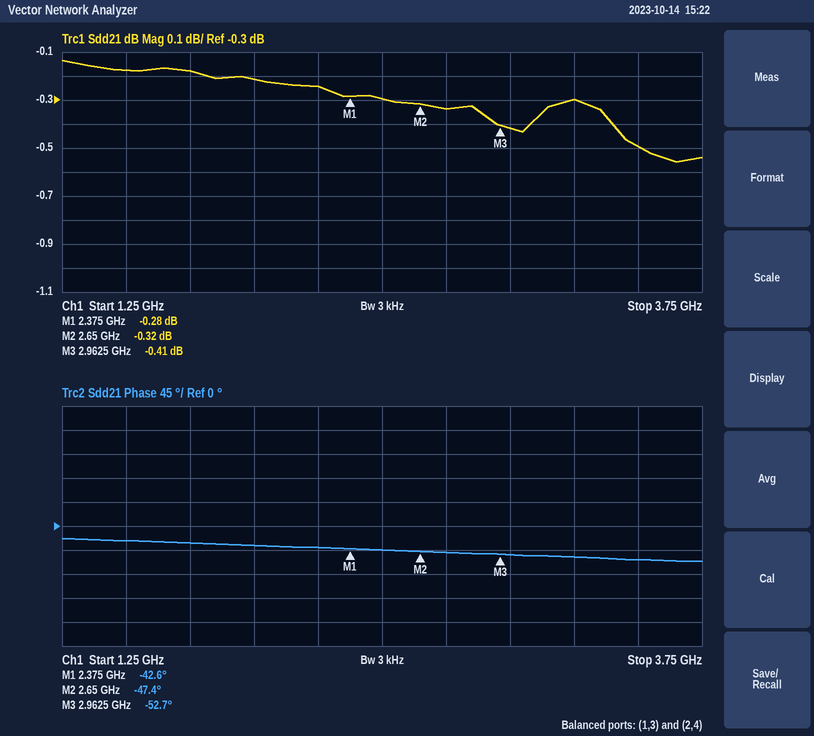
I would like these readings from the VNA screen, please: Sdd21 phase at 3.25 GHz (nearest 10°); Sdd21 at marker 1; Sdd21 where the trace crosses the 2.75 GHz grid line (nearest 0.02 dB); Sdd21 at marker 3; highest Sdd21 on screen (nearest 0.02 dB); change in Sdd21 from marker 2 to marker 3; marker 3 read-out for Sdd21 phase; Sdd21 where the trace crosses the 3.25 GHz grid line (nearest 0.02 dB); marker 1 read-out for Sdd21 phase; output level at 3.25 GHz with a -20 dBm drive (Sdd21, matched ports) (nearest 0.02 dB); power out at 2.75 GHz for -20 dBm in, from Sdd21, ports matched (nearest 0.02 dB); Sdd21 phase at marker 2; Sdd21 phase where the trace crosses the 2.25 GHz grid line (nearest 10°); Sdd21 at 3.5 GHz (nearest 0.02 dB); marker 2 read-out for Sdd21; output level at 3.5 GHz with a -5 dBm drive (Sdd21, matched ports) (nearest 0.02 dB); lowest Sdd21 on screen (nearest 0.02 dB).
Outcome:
-60°
-0.28 dB
-0.34 dB
-0.41 dB
-0.14 dB
-0.09 dB
-52.7°
-0.30 dB
-42.6°
-20.30 dBm
-20.34 dBm
-47.4°
-40°
-0.50 dB
-0.32 dB
-5.50 dBm
-0.56 dB
